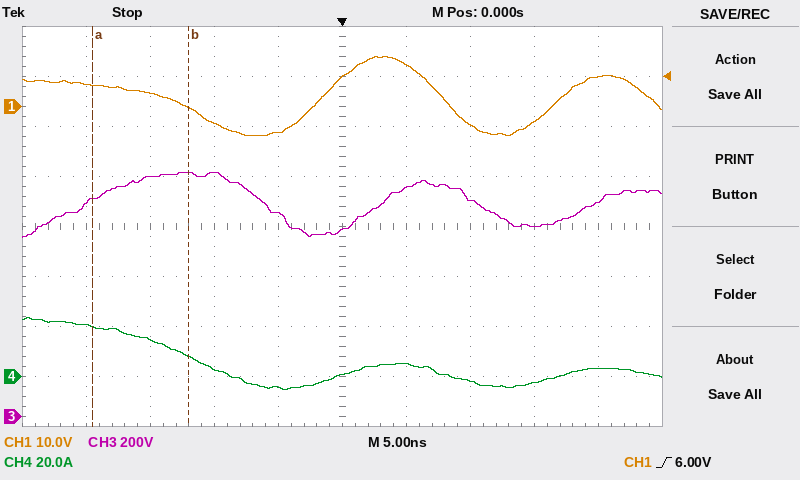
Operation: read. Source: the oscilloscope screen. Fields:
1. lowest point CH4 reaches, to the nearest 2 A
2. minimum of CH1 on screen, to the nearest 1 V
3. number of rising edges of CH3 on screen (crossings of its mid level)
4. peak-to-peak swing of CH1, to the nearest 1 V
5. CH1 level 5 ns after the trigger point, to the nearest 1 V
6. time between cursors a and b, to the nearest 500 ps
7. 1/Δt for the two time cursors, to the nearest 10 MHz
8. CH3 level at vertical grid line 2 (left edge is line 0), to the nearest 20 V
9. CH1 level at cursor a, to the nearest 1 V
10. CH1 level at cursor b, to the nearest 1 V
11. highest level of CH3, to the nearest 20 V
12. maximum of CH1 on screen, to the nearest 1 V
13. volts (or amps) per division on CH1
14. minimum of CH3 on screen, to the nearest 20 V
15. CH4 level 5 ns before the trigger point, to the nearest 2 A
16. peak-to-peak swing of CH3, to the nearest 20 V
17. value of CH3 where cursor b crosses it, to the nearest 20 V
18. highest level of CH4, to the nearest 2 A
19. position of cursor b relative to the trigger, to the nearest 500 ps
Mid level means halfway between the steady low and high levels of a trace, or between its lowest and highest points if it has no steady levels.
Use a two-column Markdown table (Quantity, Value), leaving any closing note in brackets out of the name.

| Quantity | Value |
|---|---|
| lowest point CH4 reaches, to the nearest 2 A | -6 A |
| minimum of CH1 on screen, to the nearest 1 V | -6 V |
| number of rising edges of CH3 on screen | 3 |
| peak-to-peak swing of CH1, to the nearest 1 V | 16 V |
| CH1 level 5 ns after the trigger point, to the nearest 1 V | 8 V |
| time between cursors a and b, to the nearest 500 ps | 7.5 ns |
| 1/Δt for the two time cursors, to the nearest 10 MHz | 130 MHz |
| CH3 level at vertical grid line 2 (left edge is line 0), to the nearest 20 V | 960 V |
| CH1 level at cursor a, to the nearest 1 V | 4 V |
| CH1 level at cursor b, to the nearest 1 V | 0 V |
| highest level of CH3, to the nearest 20 V | 980 V |
| maximum of CH1 on screen, to the nearest 1 V | 10 V |
| volts (or amps) per division on CH1 | 10 V |
| minimum of CH3 on screen, to the nearest 20 V | 720 V |
| CH4 level 5 ns before the trigger point, to the nearest 2 A | -4 A |
| peak-to-peak swing of CH3, to the nearest 20 V | 260 V |
| value of CH3 where cursor b crosses it, to the nearest 20 V | 980 V |
| highest level of CH4, to the nearest 2 A | 24 A |
| position of cursor b relative to the trigger, to the nearest 500 ps | -12.0 ns |
